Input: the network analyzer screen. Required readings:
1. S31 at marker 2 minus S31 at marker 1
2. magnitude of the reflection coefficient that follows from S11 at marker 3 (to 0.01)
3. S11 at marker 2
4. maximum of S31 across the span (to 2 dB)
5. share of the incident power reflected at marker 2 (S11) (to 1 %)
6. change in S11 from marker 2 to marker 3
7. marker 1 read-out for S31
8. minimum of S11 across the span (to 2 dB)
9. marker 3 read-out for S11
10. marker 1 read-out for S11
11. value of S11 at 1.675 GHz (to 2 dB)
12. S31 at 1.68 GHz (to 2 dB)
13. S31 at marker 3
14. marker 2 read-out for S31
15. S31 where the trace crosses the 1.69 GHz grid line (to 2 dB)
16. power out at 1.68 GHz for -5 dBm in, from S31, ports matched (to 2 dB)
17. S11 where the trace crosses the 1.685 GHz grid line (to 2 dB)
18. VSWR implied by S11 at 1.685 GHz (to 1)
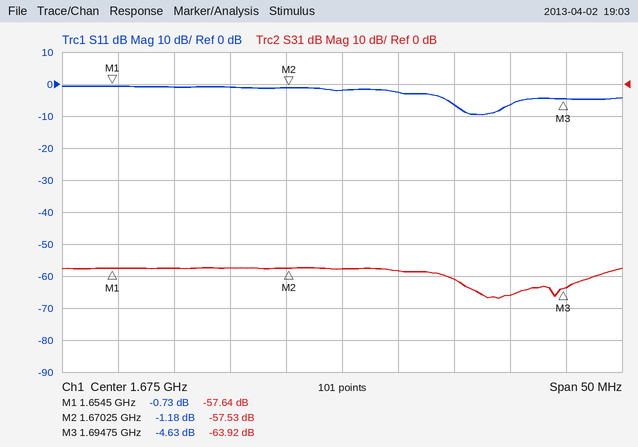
0.11 dB
0.59
-1.18 dB
-58 dB
76 %
-3.45 dB
-57.64 dB
-10 dB
-4.63 dB
-0.73 dB
-2 dB
-58 dB
-63.92 dB
-57.53 dB
-66 dB
-64 dBm
-6 dB
3
